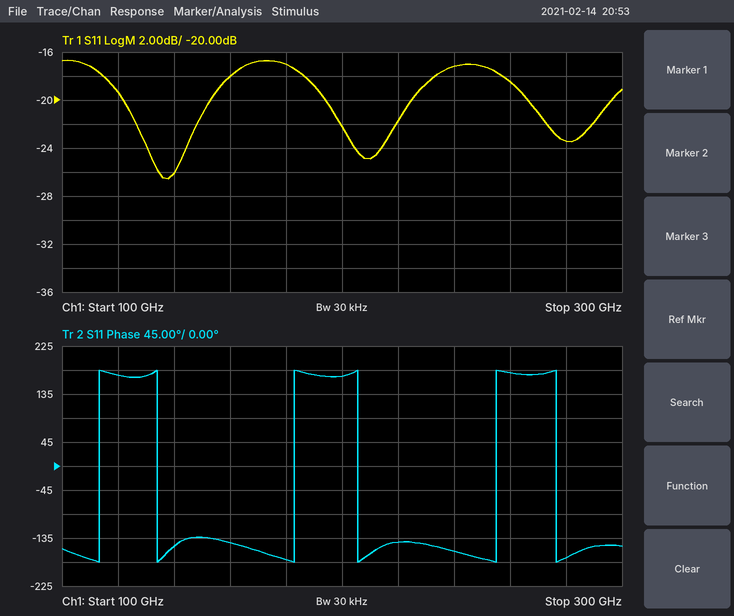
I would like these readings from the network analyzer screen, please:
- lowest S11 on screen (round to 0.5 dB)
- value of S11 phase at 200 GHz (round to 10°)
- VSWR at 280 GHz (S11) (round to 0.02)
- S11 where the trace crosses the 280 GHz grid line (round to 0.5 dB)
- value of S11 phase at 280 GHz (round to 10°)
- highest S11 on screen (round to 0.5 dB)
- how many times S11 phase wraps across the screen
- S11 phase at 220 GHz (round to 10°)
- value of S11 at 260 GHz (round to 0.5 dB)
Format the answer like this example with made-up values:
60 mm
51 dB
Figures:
-26.5 dB
170°
1.14
-23.5 dB
-170°
-16.5 dB
6
-140°
-18.5 dB
